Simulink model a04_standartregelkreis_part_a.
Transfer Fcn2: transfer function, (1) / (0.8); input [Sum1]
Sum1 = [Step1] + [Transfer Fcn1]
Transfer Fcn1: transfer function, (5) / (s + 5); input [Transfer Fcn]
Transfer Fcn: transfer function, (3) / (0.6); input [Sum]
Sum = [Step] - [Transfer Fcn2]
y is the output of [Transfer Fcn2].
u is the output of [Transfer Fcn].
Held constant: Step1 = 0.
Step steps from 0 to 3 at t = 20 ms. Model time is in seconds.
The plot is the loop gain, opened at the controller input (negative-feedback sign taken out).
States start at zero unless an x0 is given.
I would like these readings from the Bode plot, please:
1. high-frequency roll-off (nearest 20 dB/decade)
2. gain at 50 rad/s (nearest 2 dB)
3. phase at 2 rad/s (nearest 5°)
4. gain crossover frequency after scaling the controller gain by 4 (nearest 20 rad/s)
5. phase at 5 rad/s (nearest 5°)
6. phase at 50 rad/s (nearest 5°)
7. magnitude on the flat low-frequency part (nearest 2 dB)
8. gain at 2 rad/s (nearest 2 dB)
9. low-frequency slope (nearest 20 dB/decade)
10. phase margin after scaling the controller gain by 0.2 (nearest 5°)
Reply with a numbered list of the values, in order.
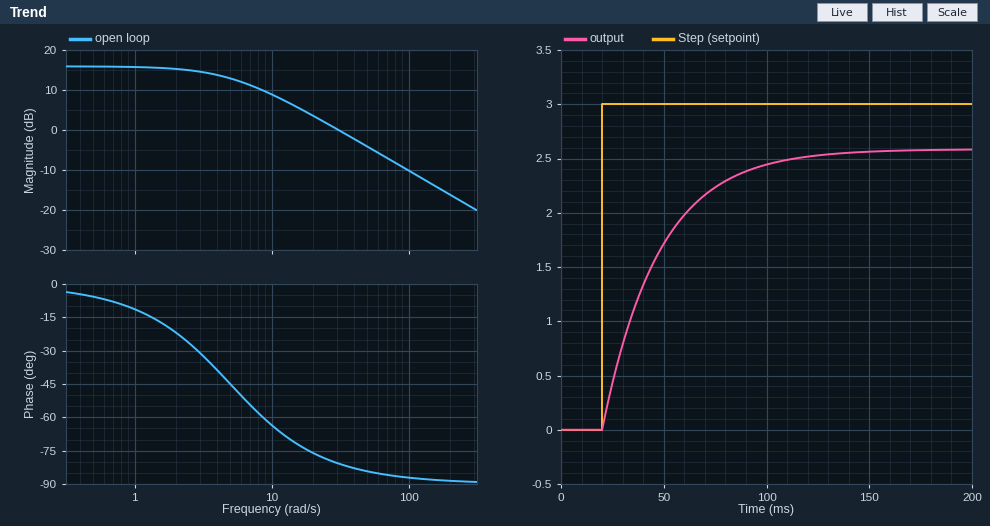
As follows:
1. -20 dB/decade
2. -4 dB
3. -20°
4. 120 rad/s
5. -45°
6. -85°
7. 16 dB
8. 16 dB
9. 0 dB/decade
10. 145°
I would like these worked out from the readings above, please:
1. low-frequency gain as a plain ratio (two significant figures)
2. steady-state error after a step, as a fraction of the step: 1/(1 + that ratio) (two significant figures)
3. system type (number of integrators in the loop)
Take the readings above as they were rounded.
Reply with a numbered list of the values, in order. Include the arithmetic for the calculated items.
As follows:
1. 10^(16 / 20) = 6.3
2. 1 / (1 + 6.3) = 0.14
3. 0
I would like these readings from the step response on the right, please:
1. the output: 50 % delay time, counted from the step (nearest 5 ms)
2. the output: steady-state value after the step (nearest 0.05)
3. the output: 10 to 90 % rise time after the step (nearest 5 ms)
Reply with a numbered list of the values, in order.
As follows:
1. 20 ms
2. 2.60
3. 60 ms
